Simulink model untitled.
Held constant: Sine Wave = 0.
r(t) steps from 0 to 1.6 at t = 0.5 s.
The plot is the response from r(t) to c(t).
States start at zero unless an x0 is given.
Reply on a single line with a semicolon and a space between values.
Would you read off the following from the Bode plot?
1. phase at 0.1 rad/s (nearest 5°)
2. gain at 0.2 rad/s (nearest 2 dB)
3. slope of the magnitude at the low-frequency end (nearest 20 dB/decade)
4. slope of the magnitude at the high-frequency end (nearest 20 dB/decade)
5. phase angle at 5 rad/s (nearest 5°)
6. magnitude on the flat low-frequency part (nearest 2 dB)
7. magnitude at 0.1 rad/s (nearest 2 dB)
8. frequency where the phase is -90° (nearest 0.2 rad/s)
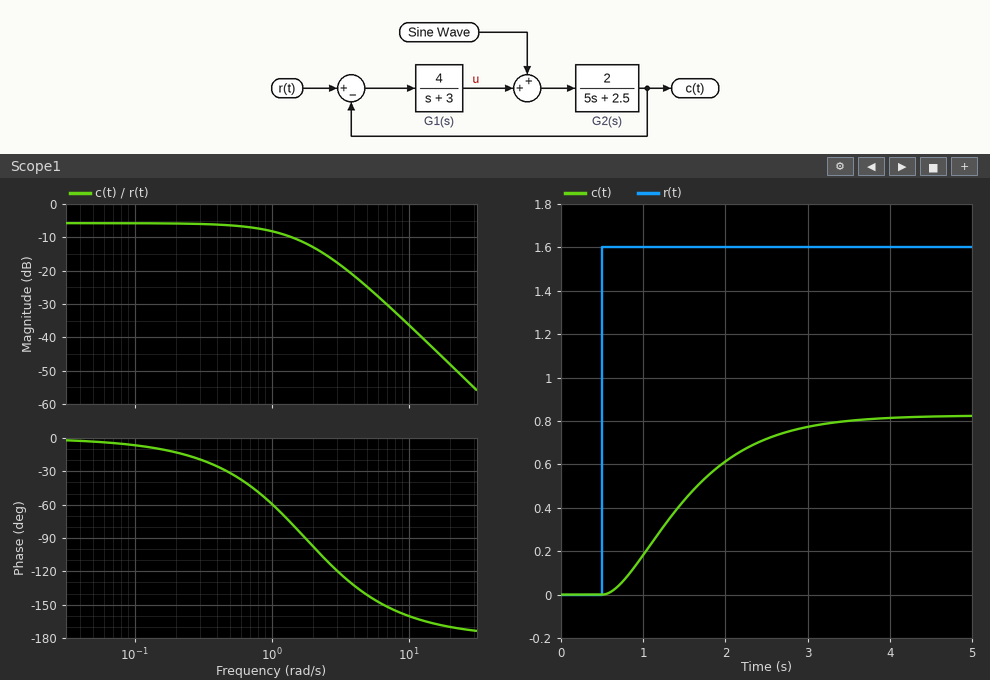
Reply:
-5°; -6 dB; 0 dB/decade; -40 dB/decade; -140°; -6 dB; -6 dB; 1.8 rad/s
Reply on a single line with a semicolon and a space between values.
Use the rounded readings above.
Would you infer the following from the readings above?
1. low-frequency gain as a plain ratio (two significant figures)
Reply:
0.50
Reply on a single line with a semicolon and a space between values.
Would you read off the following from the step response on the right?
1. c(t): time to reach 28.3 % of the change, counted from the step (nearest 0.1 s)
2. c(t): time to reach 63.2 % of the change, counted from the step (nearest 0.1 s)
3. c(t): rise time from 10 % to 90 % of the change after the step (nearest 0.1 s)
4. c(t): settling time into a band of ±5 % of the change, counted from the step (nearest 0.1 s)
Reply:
0.6 s; 1.2 s; 1.9 s; 2.7 s
